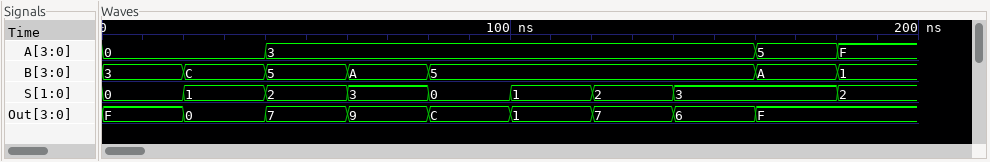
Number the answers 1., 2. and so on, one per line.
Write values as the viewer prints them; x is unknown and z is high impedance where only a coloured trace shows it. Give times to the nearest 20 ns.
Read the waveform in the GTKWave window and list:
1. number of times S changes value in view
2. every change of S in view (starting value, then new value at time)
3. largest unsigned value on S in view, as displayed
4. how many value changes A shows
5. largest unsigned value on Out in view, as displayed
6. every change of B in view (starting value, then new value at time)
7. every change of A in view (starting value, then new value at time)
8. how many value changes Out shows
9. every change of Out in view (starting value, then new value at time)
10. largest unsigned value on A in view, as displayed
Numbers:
1. 8
2. 0, 1 at 20 ns, 2 at 40 ns, 3 at 60 ns, 0 at 80 ns, 1 at 100 ns, 2 at 120 ns, 3 at 140 ns, 2 at 180 ns
3. 3
4. 3
5. F
6. 3, C at 20 ns, 5 at 40 ns, A at 60 ns, 5 at 80 ns, A at 160 ns, 1 at 180 ns
7. 0, 3 at 40 ns, 5 at 160 ns, F at 180 ns
8. 8
9. F, 0 at 20 ns, 7 at 40 ns, 9 at 60 ns, C at 80 ns, 1 at 100 ns, 7 at 120 ns, 6 at 140 ns, F at 160 ns
10. F
